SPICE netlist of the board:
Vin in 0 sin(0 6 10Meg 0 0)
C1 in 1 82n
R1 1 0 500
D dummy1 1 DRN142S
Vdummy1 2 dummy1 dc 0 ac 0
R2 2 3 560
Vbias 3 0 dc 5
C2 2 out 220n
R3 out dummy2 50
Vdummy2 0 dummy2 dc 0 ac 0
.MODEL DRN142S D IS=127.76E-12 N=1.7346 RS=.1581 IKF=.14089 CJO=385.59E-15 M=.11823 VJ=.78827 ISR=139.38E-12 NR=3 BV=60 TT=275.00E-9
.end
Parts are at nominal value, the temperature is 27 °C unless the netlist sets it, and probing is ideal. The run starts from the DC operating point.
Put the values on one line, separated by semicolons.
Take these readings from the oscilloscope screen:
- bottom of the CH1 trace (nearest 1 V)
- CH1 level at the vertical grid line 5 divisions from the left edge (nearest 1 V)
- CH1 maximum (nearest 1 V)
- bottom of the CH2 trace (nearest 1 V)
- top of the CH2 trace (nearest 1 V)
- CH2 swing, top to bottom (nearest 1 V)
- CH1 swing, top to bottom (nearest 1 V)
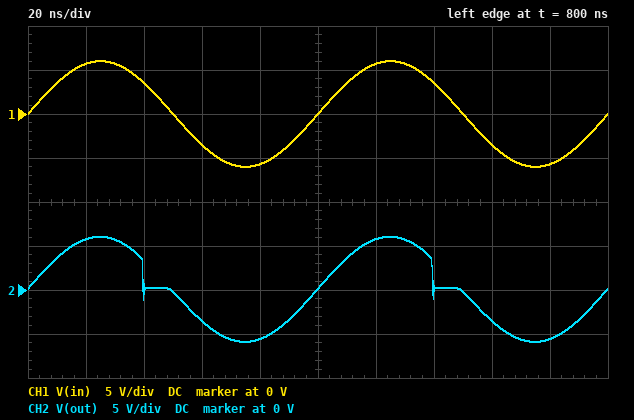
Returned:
-6 V; 0 V; 6 V; -6 V; 6 V; 12 V; 12 V
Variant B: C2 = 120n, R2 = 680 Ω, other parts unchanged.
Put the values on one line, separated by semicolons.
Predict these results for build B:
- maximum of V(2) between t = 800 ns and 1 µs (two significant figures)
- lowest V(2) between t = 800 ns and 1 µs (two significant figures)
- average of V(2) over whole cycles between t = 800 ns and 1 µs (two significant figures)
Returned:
8.6 V; -3.3 V; 2.4 V
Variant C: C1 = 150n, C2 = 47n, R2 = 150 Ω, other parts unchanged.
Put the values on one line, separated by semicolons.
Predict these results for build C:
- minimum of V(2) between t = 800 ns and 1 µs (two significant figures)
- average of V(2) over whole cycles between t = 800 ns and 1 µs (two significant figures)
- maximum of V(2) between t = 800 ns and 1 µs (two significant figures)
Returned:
-1.9 V; 3.9 V; 10 V
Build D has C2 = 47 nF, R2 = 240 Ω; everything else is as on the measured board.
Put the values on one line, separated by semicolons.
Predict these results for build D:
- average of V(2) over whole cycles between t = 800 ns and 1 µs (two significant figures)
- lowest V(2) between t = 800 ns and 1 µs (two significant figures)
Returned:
3.5 V; -2.3 V
